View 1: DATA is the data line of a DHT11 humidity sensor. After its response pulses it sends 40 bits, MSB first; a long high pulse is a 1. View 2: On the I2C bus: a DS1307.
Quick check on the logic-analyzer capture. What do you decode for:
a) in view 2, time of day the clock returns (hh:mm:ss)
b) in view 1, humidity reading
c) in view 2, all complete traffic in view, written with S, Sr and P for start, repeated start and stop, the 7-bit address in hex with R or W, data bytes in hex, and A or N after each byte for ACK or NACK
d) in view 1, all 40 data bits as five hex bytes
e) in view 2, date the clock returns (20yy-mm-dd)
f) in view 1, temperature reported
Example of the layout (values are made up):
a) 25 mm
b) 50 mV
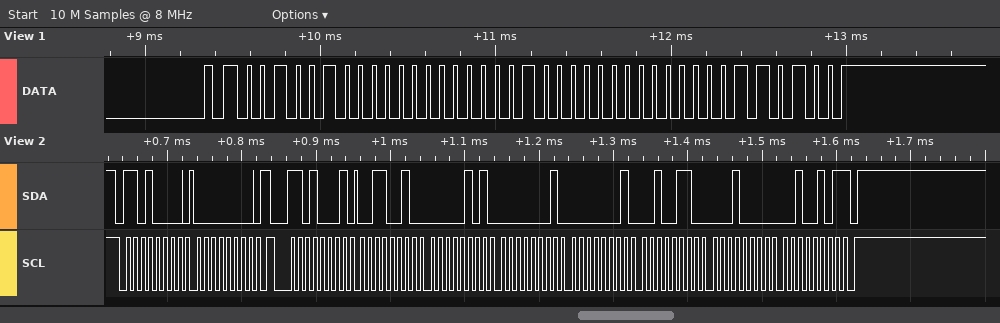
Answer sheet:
a) 01:05:32
b) 36 %
c) S 68W A 00 A Sr 68R A 32 A 05 A 01 A 01 A 26 A 10 A 25 N P
d) 24 00 10 00 34
e) 2025-10-26
f) 16.0 °C
